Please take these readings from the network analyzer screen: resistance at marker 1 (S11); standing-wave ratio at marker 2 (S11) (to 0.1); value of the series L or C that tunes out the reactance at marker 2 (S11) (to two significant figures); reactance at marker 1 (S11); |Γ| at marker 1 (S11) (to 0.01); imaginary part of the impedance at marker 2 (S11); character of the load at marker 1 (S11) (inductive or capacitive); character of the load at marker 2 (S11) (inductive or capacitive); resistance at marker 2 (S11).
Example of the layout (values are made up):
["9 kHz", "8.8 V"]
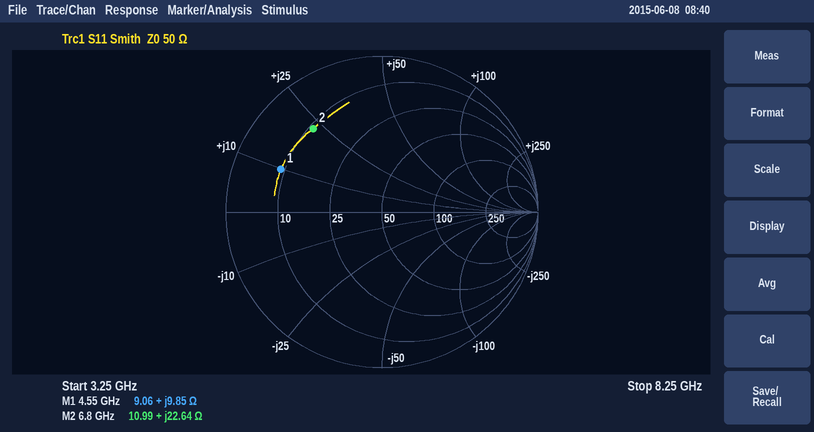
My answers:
["9.06 Ω", "5.5", "1.0 pF", "+9.85 Ω", "0.70", "+22.64 Ω", "inductive", "inductive", "10.99 Ω"]
